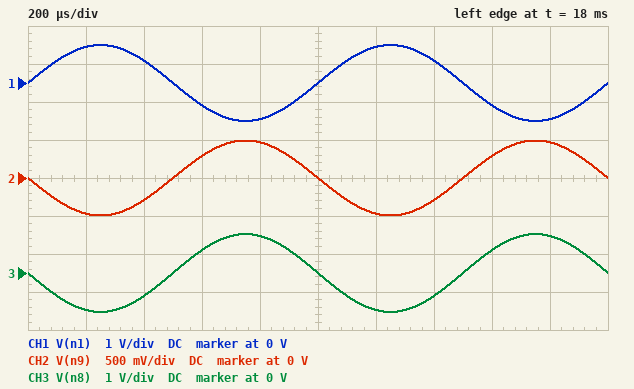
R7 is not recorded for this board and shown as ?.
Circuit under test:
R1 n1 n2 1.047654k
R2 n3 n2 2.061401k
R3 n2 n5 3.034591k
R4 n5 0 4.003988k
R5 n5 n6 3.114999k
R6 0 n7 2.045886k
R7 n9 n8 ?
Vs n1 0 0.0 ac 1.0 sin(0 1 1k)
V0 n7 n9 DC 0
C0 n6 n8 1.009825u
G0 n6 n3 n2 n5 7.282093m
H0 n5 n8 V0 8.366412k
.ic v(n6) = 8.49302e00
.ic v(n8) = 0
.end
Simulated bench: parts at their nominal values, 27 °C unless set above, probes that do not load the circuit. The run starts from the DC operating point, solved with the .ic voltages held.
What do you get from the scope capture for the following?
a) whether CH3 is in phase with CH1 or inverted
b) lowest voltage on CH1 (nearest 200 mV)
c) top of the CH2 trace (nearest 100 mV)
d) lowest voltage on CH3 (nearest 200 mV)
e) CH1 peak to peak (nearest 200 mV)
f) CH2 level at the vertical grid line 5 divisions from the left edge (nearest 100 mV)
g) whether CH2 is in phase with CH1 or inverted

inverted
-1.0 V
500 mV
-1.0 V
2.0 V
0 V
inverted
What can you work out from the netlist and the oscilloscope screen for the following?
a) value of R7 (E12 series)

2.2 kΩ
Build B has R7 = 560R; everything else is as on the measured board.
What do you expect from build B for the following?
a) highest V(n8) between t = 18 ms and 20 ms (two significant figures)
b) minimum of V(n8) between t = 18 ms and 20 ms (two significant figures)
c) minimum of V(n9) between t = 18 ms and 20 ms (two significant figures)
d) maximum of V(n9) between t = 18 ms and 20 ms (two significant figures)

420 mV
-420 mV
-330 mV
330 mV
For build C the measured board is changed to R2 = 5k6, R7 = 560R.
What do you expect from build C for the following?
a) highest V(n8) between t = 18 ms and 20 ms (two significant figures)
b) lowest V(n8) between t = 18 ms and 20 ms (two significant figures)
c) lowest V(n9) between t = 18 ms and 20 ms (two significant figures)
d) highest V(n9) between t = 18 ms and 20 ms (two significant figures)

420 mV
-420 mV
-330 mV
330 mV
